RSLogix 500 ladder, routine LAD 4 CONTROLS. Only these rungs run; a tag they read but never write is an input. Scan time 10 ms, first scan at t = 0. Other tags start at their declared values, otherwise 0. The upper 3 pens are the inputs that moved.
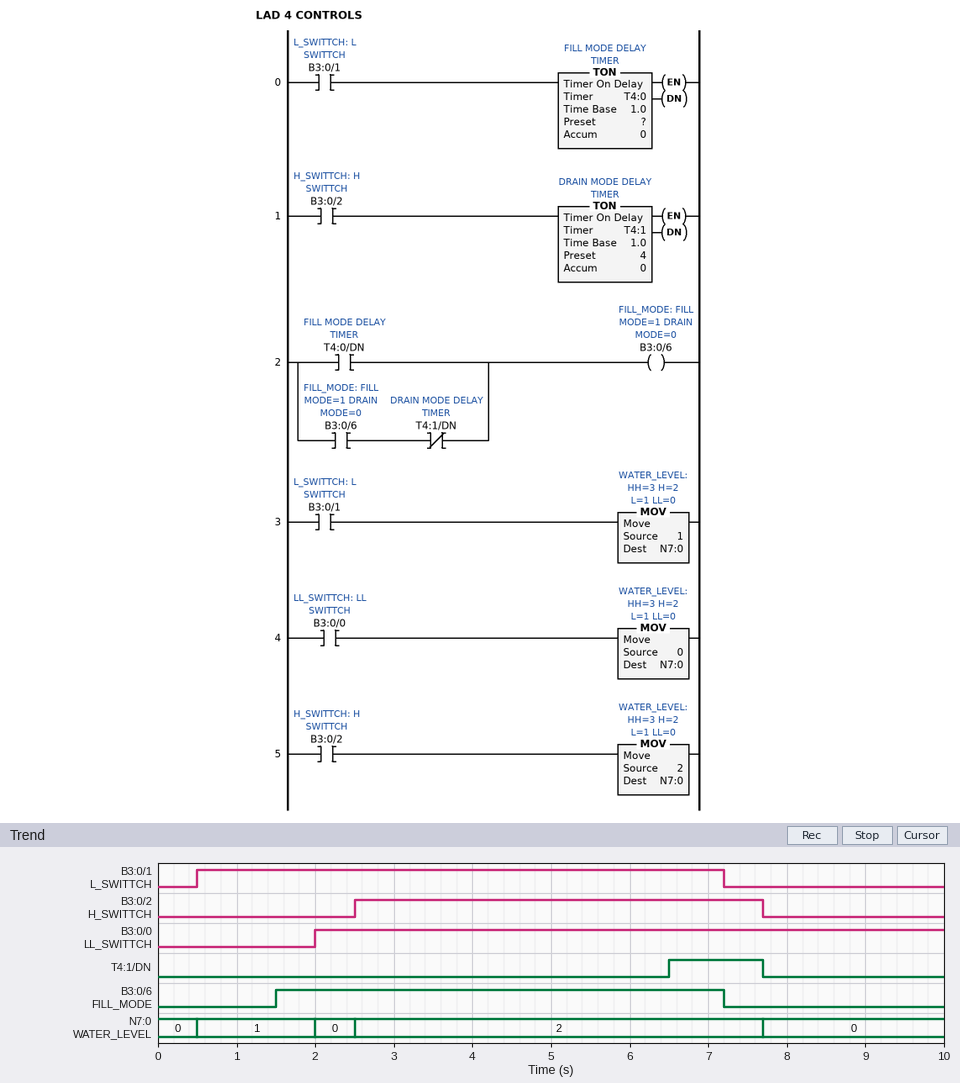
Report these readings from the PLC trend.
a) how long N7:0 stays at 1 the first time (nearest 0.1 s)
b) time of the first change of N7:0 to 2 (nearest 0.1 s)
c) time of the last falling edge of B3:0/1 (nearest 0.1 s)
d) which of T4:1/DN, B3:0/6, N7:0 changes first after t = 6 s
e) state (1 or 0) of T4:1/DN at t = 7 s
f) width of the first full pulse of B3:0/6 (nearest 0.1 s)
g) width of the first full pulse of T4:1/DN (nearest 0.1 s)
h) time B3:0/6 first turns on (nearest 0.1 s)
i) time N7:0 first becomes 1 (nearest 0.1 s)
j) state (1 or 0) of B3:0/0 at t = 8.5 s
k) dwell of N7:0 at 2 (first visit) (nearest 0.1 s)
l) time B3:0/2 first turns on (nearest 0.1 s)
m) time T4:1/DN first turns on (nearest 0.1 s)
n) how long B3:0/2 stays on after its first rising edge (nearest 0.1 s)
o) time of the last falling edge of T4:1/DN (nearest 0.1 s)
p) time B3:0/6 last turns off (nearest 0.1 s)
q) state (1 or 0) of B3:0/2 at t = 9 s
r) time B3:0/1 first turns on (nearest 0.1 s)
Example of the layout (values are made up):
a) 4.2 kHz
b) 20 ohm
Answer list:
a) 1.5 s
b) 2.5 s
c) 7.2 s
d) T4:1/DN
e) 1
f) 5.7 s
g) 1.2 s
h) 1.5 s
i) 0.5 s
j) 1
k) 5.2 s
l) 2.5 s
m) 6.5 s
n) 5.2 s
o) 7.7 s
p) 7.2 s
q) 0
r) 0.5 s
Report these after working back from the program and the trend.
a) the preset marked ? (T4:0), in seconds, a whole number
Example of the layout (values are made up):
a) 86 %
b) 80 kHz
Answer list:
a) 1 s
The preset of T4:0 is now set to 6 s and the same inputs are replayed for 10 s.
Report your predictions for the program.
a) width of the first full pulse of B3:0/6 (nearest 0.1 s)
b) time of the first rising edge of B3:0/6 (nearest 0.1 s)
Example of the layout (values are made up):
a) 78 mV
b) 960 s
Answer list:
a) 0.7 s
b) 6.5 s
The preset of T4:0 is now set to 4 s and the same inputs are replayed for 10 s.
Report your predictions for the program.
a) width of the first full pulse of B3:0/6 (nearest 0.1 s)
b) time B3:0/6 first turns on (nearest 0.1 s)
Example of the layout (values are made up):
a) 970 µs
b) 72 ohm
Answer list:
a) 2.7 s
b) 4.5 s
